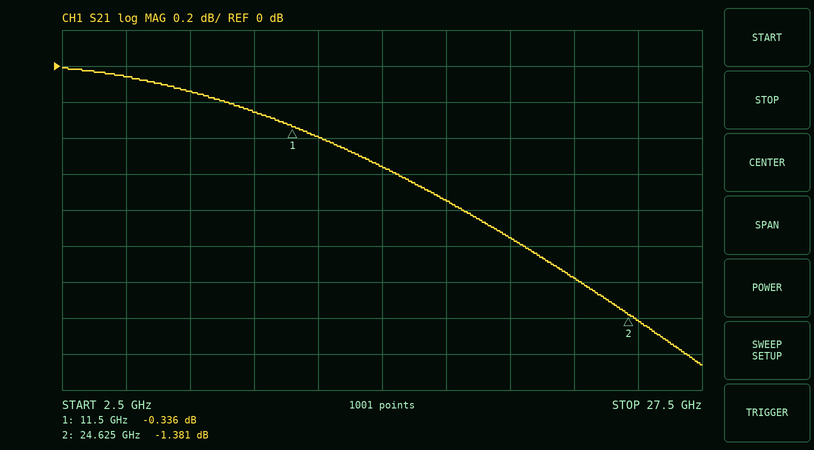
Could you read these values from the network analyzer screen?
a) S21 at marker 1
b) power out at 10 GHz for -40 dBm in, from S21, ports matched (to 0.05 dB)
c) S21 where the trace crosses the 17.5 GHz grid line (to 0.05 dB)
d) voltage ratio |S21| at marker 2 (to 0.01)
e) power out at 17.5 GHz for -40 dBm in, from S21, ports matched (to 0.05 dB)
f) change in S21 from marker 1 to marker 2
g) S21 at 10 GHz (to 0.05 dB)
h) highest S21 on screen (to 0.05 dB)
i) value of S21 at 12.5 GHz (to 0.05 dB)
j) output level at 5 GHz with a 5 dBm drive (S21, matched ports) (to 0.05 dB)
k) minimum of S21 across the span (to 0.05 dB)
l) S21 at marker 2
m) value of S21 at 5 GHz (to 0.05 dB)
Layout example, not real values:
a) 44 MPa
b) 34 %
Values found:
a) -0.336 dB
b) -40.25 dBm
c) -0.75 dB
d) 0.85
e) -40.75 dBm
f) -1.045 dB
g) -0.25 dB
h) 0.00 dB
i) -0.40 dB
j) 4.95 dBm
k) -1.65 dB
l) -1.381 dB
m) -0.05 dB
